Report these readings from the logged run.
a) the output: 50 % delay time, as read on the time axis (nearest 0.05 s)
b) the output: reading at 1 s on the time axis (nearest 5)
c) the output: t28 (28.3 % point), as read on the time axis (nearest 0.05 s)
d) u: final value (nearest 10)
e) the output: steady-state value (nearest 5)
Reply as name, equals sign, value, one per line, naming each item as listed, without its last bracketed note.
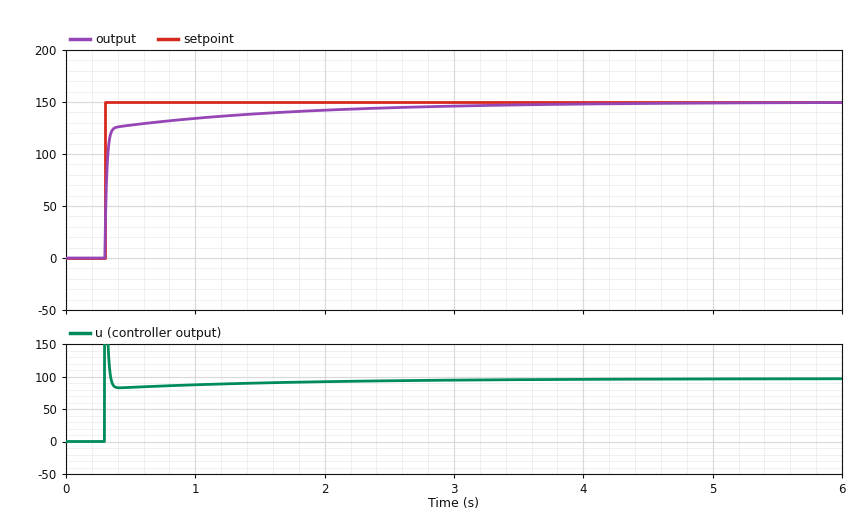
the output: 50 % delay time, as read on the time axis = 0.30 s
the output: reading at 1 s on the time axis = 135
the output: t28 (28.3 % point), as read on the time axis = 0.30 s
u: final value = 100
the output: steady-state value = 150
